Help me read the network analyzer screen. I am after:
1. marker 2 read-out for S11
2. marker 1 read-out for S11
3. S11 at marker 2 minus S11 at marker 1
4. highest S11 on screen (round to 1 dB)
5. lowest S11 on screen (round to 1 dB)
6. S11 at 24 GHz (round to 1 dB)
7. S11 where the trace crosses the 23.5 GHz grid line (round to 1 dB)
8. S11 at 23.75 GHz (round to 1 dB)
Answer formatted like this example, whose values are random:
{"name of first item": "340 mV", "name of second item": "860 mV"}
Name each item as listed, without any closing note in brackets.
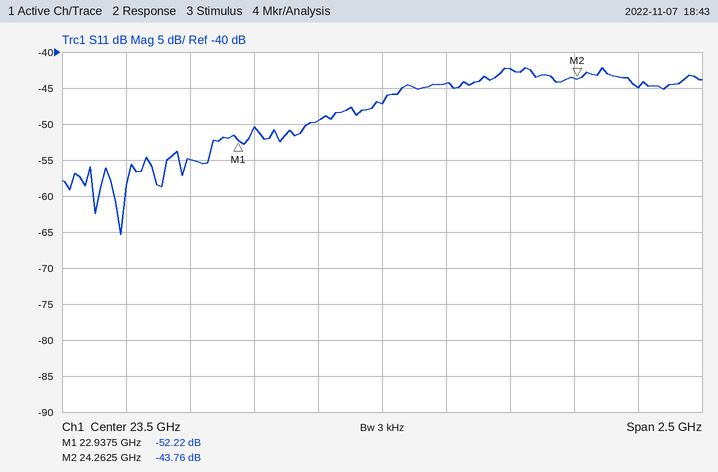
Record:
{"marker 2 read-out for S11": "-43.76 dB", "marker 1 read-out for S11": "-52.22 dB", "S11 at marker 2 minus S11 at marker 1": "8.46 dB", "highest S11 on screen": "-42 dB", "lowest S11 on screen": "-65 dB", "S11 at 24 GHz": "-42 dB", "S11 where the trace crosses the 23.5 GHz grid line": "-47 dB", "S11 at 23.75 GHz": "-44 dB"}
